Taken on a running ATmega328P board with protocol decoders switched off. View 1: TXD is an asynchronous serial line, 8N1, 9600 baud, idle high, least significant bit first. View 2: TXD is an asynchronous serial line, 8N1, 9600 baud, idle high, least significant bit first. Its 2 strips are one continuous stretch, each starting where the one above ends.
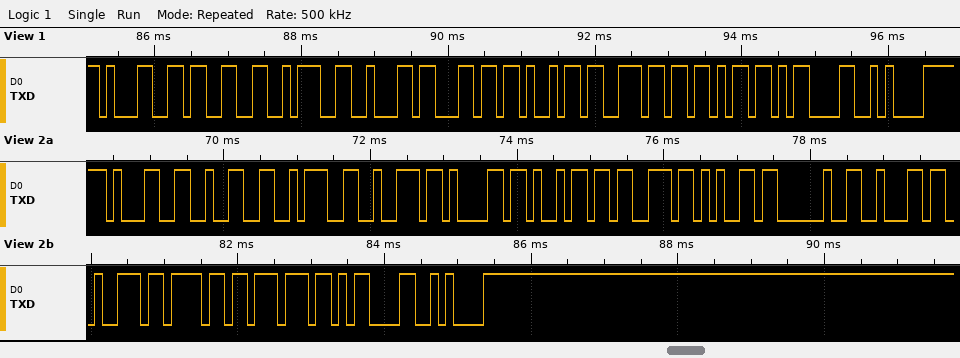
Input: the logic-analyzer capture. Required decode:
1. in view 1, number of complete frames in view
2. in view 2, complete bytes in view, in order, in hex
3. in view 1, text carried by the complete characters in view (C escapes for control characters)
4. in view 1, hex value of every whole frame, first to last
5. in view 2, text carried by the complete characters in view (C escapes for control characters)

10
0x31 0x32 0x3A 0x72 0x61 0x69 0x73 0x65 0x20 0x62 0x72 0x6F 0x77 0x0D 0x0A
"13:blink\r\n"
31 33 3A 62 6C 69 6E 6B 0D 0A
"12:raise brow\r\n"
